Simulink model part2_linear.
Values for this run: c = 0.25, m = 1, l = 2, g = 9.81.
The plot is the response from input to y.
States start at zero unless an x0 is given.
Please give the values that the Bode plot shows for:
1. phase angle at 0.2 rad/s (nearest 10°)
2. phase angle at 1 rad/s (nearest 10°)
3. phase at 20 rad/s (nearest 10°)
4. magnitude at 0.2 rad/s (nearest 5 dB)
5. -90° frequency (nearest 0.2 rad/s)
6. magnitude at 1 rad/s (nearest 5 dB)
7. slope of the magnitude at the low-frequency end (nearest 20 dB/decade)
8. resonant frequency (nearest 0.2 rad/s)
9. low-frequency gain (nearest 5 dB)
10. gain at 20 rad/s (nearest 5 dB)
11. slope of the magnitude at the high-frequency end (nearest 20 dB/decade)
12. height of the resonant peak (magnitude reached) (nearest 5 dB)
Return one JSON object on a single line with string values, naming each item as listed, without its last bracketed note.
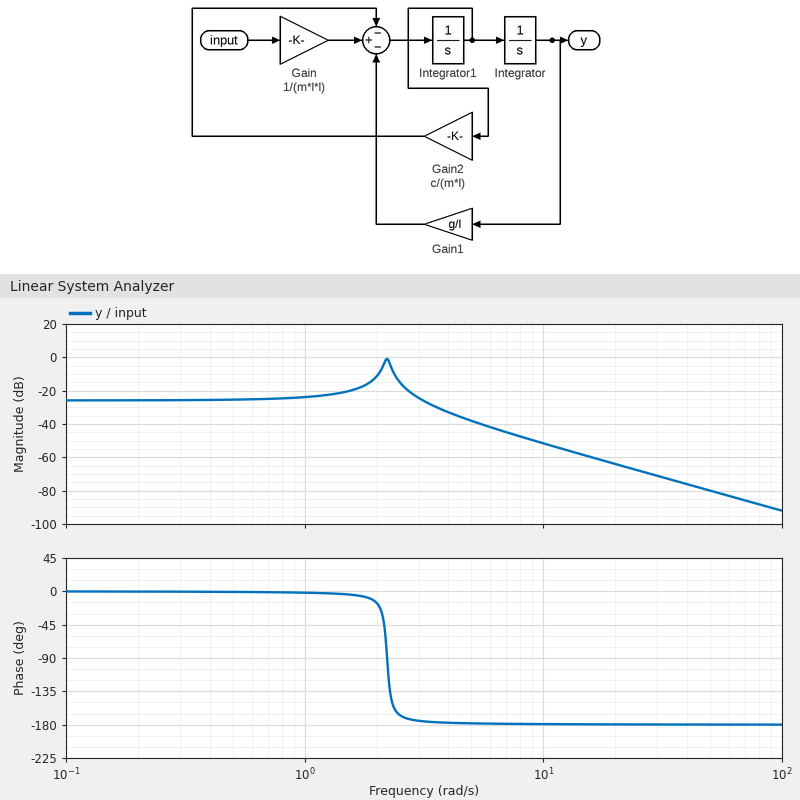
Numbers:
{"phase angle at 0.2 rad/s": "0°", "phase angle at 1 rad/s": "0°", "phase at 20 rad/s": "-180°", "magnitude at 0.2 rad/s": "-25 dB", "-90° frequency": "2.2 rad/s", "magnitude at 1 rad/s": "-25 dB", "slope of the magnitude at the low-frequency end": "0 dB/decade", "resonant frequency": "2.2 rad/s", "low-frequency gain": "-25 dB", "gain at 20 rad/s": "-65 dB", "slope of the magnitude at the high-frequency end": "-40 dB/decade", "height of the resonant peak (magnitude reached)": "0 dB"}
